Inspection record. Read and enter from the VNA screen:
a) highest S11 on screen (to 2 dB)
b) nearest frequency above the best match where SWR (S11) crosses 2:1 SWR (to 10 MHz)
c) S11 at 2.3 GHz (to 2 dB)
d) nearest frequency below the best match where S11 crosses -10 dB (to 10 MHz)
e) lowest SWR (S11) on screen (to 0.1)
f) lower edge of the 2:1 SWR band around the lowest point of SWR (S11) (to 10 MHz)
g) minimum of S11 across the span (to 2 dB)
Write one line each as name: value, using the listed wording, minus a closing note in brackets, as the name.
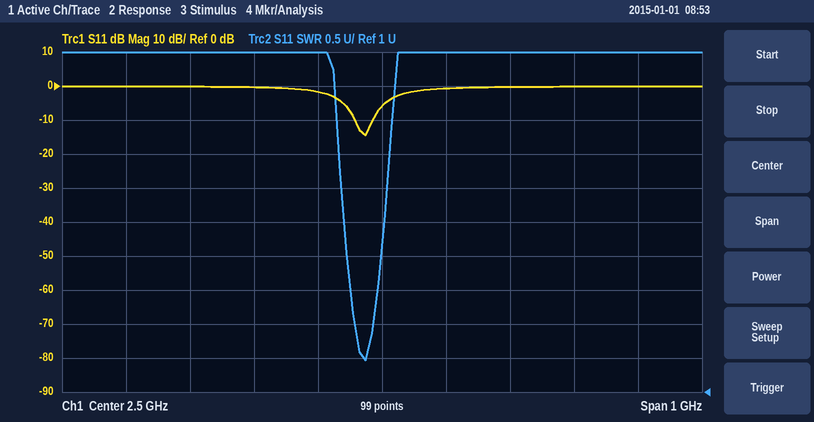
highest S11 on screen: 0 dB
nearest frequency above the best match where SWR (S11) crosses 2:1 SWR: 2.49 GHz
S11 at 2.3 GHz: 0 dB
nearest frequency below the best match where S11 crosses -10 dB: 2.46 GHz
lowest SWR (S11) on screen: 1.5
lower edge of the 2:1 SWR band around the lowest point of SWR (S11): 2.46 GHz
minimum of S11 across the span: -14 dB
